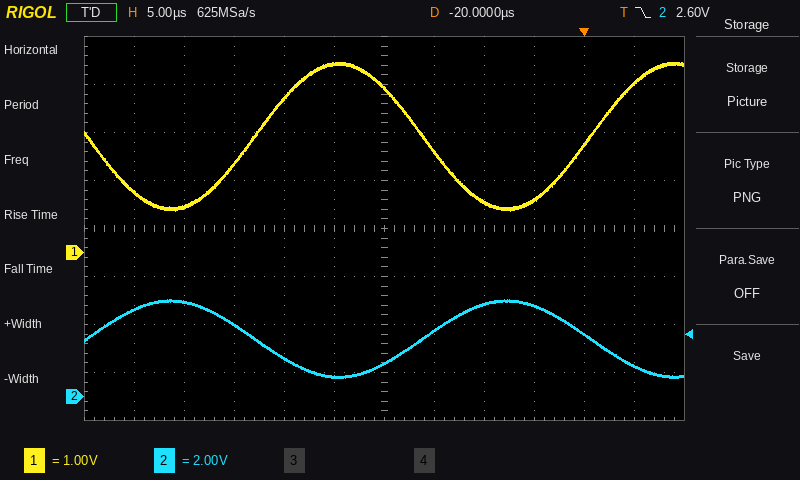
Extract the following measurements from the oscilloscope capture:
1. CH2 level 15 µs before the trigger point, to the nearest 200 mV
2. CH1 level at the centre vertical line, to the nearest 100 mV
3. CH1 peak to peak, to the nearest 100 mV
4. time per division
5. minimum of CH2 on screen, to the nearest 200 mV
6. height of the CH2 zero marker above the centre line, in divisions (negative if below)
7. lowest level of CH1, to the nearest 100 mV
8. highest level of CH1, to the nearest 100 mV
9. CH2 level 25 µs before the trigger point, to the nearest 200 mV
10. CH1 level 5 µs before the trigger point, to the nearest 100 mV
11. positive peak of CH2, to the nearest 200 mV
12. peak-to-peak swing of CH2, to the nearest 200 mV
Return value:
2.8 V
3.4 V
3.1 V
5 µs
800 mV
-3.5 div
900 mV
4.0 V
800 mV
1.1 V
4.0 V
3.2 V
